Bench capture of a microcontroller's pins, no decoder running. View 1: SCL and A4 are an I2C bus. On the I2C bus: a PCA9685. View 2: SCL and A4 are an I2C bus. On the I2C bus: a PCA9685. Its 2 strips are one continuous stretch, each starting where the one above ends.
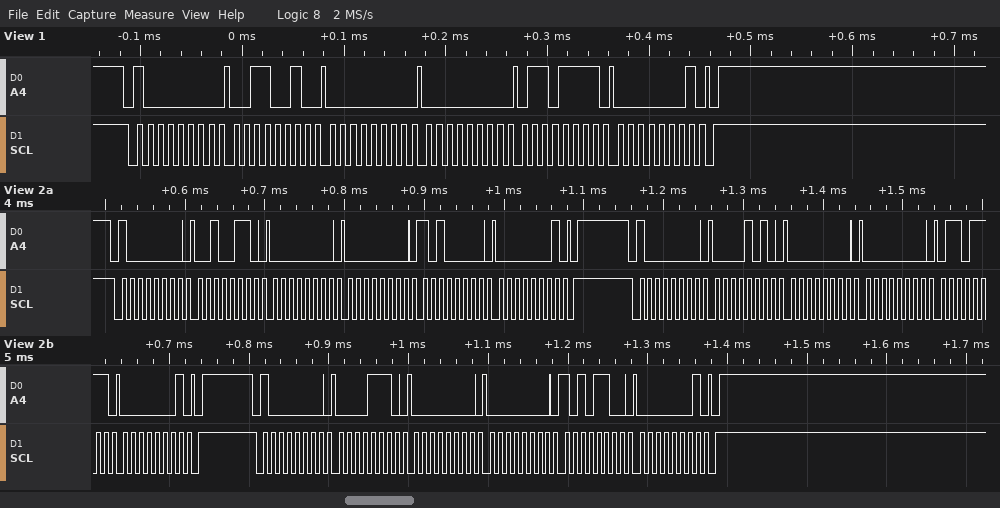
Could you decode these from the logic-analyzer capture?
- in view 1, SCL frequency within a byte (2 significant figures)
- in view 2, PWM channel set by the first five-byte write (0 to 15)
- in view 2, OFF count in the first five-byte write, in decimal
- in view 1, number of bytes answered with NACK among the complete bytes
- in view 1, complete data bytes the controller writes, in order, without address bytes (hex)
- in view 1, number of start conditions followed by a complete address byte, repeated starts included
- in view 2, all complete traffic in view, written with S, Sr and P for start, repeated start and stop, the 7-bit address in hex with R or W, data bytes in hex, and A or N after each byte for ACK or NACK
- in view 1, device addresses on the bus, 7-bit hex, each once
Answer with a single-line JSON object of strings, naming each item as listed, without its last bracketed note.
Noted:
{"in view 1, SCL frequency within a byte": "100 kHz", "in view 2, PWM channel set by the first five-byte write": "8", "in view 2, OFF count in the first five-byte write, in decimal": "416", "in view 1, number of bytes answered with NACK among the complete bytes": "0", "in view 1, complete data bytes the controller writes, in order, without address bytes": "32 00 00 6F 01", "in view 1, number of start conditions followed by a complete address byte, repeated starts included": "1", "in view 2, all complete traffic in view, written with S, Sr and P for start, repeated start and stop, the 7-bit address in hex with R or W, data bytes in hex, and A or N after each byte for ACK or NACK": "S 40W A 26 A 00 A 00 A A0 A 01 A P S 40W A 0A A 00 A 00 A 6F A 01 A P S 40W A 0E A 00 A 00 A AC A 01 A P", "in view 1, device addresses on the bus, 7-bit hex, each once": "0x40"}
